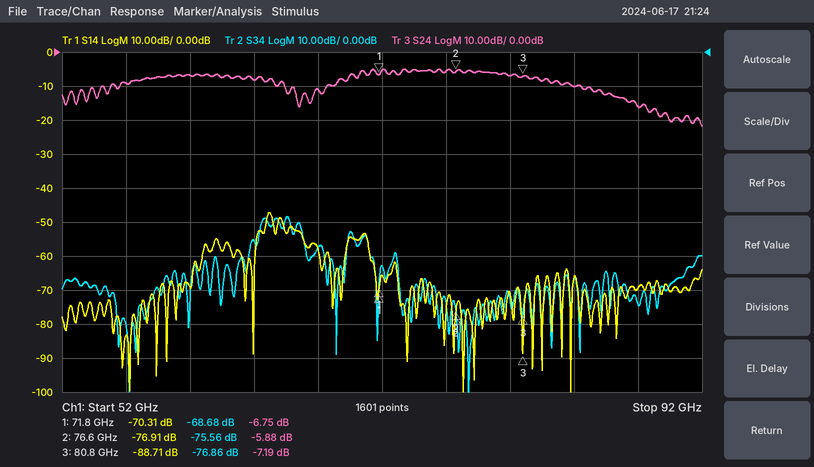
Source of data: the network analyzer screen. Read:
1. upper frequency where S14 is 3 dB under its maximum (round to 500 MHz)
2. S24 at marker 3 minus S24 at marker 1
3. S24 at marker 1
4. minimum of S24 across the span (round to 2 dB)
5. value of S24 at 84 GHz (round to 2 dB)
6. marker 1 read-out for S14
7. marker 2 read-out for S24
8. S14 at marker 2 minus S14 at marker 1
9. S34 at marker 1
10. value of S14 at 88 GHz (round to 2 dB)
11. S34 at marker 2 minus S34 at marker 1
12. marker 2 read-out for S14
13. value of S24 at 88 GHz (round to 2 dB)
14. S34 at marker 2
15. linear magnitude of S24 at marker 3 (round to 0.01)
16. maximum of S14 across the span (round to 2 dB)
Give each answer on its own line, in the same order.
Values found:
65.0 GHz
-0.44 dB
-6.75 dB
-22 dB
-10 dB
-70.31 dB
-5.88 dB
-6.60 dB
-68.68 dB
-70 dB
-6.88 dB
-76.91 dB
-16 dB
-75.56 dB
0.44
-48 dB
